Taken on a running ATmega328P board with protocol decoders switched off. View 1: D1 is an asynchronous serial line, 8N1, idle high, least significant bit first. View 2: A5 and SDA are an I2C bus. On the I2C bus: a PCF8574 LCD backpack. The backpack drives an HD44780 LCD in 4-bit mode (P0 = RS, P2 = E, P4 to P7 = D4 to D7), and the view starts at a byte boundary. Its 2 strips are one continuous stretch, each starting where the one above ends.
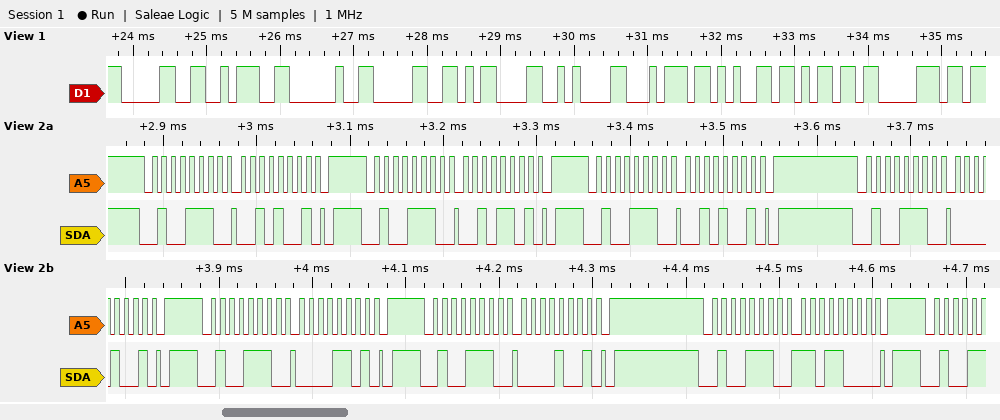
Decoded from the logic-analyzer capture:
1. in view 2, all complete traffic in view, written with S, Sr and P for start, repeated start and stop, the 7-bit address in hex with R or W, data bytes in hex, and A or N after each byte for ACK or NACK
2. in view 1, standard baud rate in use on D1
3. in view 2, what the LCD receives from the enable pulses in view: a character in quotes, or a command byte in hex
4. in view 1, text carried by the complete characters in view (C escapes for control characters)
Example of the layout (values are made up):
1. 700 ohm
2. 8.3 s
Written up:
1. S 27W A 29 A P S 27W A 2D A P S 27W A 29 A P S 27W A 09 A P S 27W A 0D A P S 27W A 09 A P S 27W A D8 A P
2. 9600 baud
3. ' '
4. "0: 0\r\ntemp"
